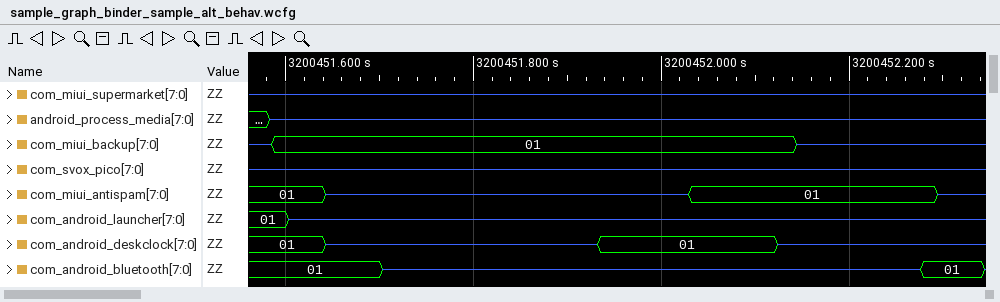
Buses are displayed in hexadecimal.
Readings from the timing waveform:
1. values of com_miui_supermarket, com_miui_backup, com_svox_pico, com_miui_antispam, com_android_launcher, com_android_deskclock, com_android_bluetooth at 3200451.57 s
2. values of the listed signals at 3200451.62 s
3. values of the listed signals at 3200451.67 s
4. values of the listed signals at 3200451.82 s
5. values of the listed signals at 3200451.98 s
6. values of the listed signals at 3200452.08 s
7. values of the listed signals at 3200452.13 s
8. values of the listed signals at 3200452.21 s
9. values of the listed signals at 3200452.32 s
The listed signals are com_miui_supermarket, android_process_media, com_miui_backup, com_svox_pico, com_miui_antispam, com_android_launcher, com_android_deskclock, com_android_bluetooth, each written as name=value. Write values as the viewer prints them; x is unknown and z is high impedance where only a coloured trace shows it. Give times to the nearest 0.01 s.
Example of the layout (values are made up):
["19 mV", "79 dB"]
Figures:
["com_miui_supermarket=z, com_miui_backup=z, com_svox_pico=z, com_miui_antispam=01, com_android_launcher=01, com_android_deskclock=01, com_android_bluetooth=01", "com_miui_supermarket=z, android_process_media=z, com_miui_backup=01, com_svox_pico=z, com_miui_antispam=01, com_android_launcher=z, com_android_deskclock=01, com_android_bluetooth=01", "com_miui_supermarket=z, android_process_media=z, com_miui_backup=01, com_svox_pico=z, com_miui_antispam=z, com_android_launcher=z, com_android_deskclock=z, com_android_bluetooth=01", "com_miui_supermarket=z, android_process_media=z, com_miui_backup=01, com_svox_pico=z, com_miui_antispam=z, com_android_launcher=z, com_android_deskclock=z, com_android_bluetooth=z", "com_miui_supermarket=z, android_process_media=z, com_miui_backup=01, com_svox_pico=z, com_miui_antispam=z, com_android_launcher=z, com_android_deskclock=01, com_android_bluetooth=z", "com_miui_supermarket=z, android_process_media=z, com_miui_backup=01, com_svox_pico=z, com_miui_antispam=01, com_android_launcher=z, com_android_deskclock=01, com_android_bluetooth=z", "com_miui_supermarket=z, android_process_media=z, com_miui_backup=01, com_svox_pico=z, com_miui_antispam=01, com_android_launcher=z, com_android_deskclock=z, com_android_bluetooth=z", "com_miui_supermarket=z, android_process_media=z, com_miui_backup=z, com_svox_pico=z, com_miui_antispam=01, com_android_launcher=z, com_android_deskclock=z, com_android_bluetooth=z", "com_miui_supermarket=z, android_process_media=z, com_miui_backup=z, com_svox_pico=z, com_miui_antispam=z, com_android_launcher=z, com_android_deskclock=z, com_android_bluetooth=01"]
